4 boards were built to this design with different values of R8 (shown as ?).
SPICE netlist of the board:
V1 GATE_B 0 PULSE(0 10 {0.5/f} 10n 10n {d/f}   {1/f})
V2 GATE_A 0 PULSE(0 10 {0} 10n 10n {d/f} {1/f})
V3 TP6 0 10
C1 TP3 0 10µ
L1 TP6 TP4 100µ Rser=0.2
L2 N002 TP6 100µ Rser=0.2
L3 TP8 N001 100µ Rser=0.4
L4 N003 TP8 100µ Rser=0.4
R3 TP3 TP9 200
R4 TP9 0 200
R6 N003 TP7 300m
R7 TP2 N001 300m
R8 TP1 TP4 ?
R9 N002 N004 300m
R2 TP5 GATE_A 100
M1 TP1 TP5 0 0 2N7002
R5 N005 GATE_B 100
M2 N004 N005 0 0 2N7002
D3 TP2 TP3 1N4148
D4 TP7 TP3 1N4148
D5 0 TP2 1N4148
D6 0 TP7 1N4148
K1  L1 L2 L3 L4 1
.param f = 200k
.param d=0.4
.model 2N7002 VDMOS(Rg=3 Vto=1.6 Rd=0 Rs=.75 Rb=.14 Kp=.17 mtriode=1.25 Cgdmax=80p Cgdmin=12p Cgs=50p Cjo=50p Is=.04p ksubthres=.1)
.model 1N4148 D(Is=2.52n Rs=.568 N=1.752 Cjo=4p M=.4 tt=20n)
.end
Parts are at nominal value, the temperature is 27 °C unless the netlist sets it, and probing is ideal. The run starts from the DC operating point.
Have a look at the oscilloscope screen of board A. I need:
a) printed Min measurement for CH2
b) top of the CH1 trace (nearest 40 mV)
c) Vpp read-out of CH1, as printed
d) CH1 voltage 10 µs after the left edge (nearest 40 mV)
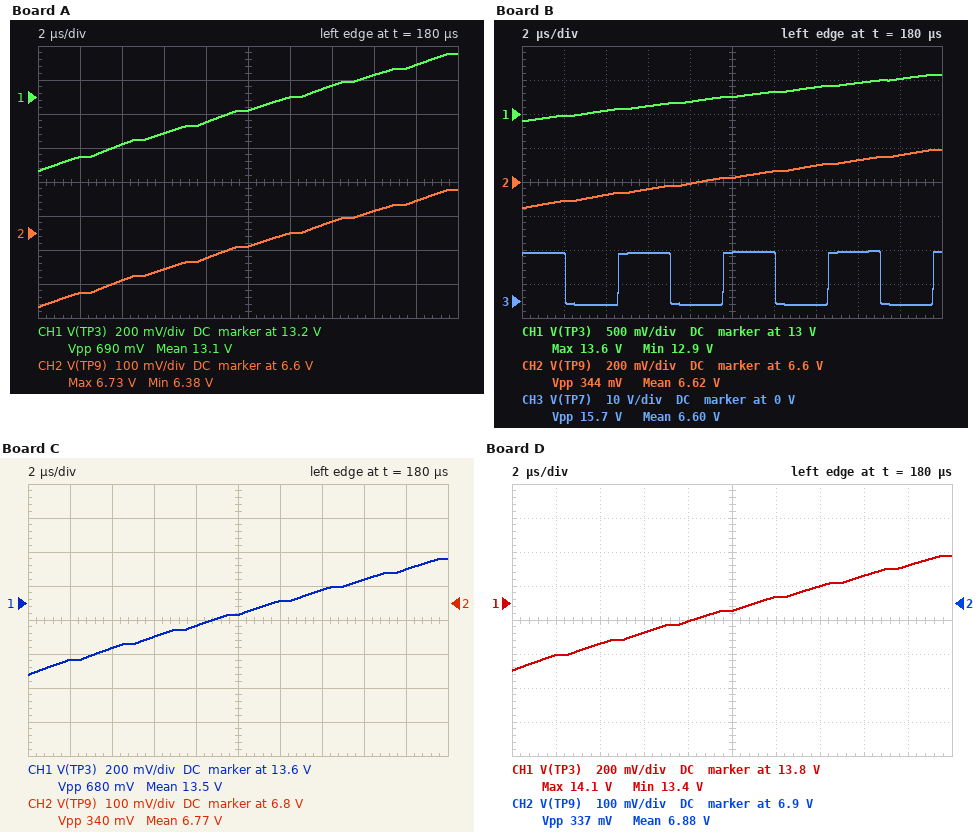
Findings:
6.38 V
13.44 V
690 mV
13.12 V
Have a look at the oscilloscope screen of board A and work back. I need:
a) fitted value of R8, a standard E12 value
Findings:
0.82 Ω
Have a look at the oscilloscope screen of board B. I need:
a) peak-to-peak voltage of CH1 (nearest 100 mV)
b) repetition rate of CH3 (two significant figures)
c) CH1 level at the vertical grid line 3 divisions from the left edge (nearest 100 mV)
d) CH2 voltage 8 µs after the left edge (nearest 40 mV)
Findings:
700 mV
200 kHz
13.1 V
6.60 V
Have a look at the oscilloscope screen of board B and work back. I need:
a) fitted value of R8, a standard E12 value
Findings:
0.68 Ω
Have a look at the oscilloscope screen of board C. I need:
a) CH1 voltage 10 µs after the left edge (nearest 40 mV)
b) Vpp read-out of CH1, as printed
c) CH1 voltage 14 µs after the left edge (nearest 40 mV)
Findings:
13.52 V
680 mV
13.68 V
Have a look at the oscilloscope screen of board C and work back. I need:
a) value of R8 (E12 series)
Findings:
0.39 Ω
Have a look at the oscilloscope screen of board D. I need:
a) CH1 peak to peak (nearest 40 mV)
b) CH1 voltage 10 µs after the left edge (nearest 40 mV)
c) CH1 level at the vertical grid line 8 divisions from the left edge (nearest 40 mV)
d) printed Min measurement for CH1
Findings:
680 mV
13.76 V
13.96 V
13.4 V
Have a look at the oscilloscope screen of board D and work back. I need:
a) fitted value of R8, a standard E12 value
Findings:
0.18 Ω
